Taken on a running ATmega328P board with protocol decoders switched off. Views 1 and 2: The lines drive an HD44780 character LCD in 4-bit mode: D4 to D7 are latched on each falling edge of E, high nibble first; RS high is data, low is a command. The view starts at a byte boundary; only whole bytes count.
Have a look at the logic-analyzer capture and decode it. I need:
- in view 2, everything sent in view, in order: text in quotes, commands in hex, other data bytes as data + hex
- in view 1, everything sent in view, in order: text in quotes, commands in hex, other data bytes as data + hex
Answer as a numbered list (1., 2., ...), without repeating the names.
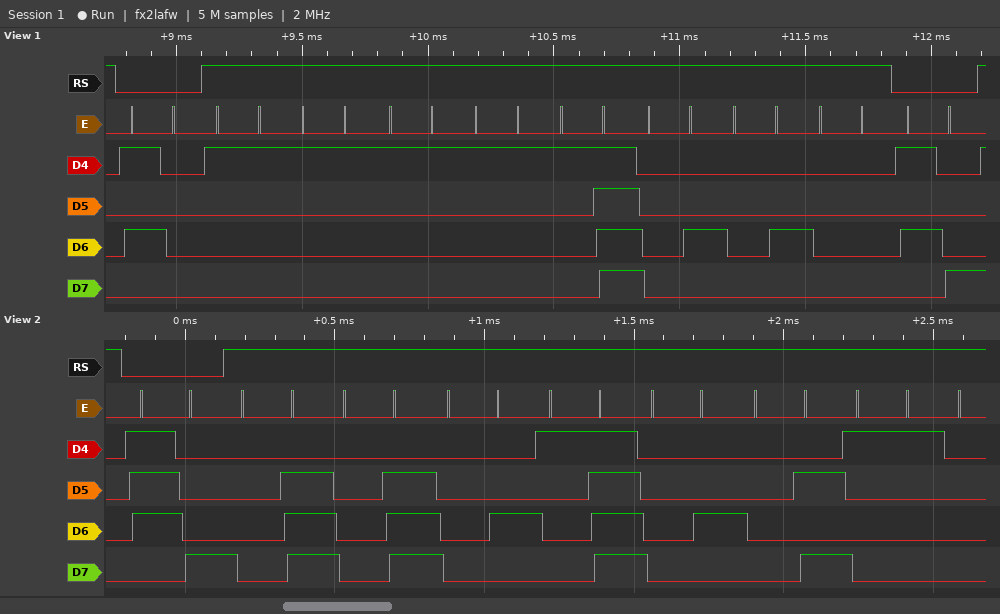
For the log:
1. 0x78 data 0E 0E 04 1F 04 0A 11
2. 0x50 data 11 11 11 11 1F 04 04 00 0x58
